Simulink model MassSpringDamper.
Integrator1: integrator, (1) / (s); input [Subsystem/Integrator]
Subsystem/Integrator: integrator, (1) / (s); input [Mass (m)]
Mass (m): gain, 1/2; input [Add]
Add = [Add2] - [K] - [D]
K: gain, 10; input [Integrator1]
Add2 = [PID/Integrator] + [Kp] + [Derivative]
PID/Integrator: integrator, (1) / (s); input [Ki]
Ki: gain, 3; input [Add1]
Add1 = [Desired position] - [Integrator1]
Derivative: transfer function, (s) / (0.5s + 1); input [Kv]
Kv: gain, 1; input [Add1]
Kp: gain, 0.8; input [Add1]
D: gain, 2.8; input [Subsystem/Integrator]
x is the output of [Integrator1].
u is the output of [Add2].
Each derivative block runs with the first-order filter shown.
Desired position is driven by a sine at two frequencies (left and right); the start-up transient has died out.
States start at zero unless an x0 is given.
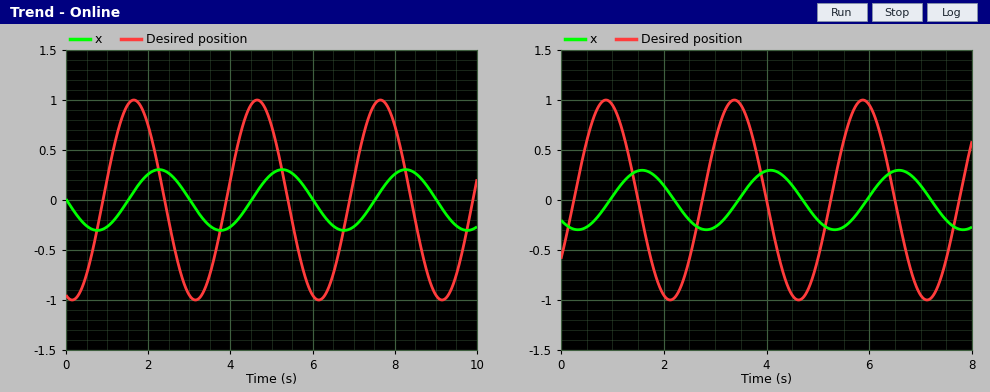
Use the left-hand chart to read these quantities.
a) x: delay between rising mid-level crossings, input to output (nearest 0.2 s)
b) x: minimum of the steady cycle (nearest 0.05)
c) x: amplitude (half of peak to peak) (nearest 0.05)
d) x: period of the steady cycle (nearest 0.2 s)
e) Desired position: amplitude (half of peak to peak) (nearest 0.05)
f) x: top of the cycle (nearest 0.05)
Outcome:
0.6 s
-0.30
0.30
3.0 s
1.00
0.30
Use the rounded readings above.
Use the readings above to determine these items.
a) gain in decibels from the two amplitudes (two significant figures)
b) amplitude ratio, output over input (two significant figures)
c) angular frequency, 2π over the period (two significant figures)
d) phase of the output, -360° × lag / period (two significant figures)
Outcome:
-10 dB
0.30
2.1 rad/s
-72°
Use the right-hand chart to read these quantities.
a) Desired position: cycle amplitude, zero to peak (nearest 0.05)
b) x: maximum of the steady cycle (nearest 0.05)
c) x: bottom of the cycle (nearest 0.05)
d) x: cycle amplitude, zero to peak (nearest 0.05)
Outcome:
1.00
0.30
-0.30
0.30
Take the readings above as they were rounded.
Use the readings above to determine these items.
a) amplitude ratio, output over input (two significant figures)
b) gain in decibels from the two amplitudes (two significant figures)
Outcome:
0.30
-10 dB
